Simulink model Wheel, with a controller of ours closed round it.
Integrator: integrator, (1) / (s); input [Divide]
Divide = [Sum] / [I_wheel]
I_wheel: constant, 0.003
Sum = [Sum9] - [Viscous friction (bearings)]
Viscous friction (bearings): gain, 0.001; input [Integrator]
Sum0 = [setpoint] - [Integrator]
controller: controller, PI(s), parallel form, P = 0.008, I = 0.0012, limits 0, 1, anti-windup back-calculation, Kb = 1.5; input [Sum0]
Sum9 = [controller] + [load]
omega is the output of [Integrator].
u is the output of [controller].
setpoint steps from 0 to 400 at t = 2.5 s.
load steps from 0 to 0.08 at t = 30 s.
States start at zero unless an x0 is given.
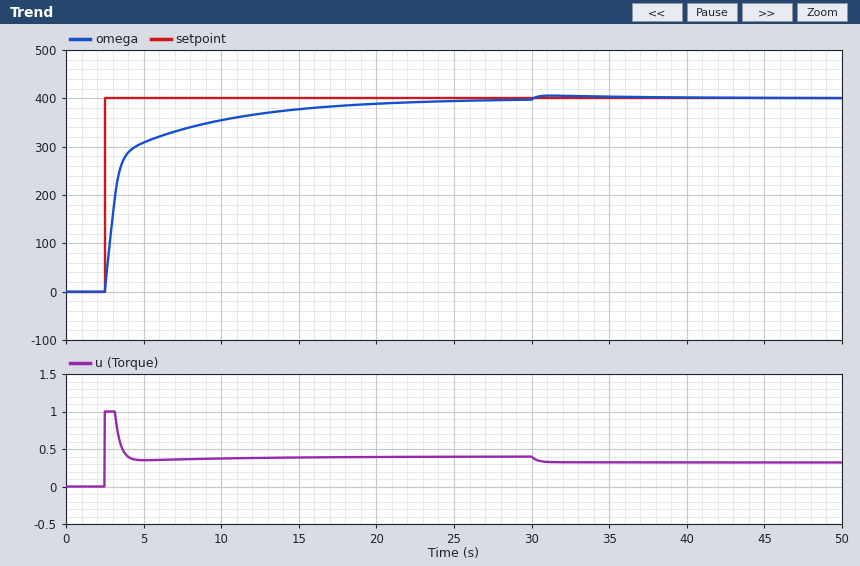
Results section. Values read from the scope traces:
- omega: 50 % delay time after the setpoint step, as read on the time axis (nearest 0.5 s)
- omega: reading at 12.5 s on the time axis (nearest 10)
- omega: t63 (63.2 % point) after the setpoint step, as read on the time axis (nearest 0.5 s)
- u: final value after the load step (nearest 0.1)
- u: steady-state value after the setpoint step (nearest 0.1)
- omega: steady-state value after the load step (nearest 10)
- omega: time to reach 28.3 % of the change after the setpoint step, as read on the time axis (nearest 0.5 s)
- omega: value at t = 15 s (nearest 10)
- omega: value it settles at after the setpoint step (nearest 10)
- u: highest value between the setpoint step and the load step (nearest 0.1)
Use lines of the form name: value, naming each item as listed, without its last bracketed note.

omega: 50 % delay time after the setpoint step, as read on the time axis: 3.0 s
omega: reading at 12.5 s on the time axis: 370
omega: t63 (63.2 % point) after the setpoint step, as read on the time axis: 3.5 s
u: final value after the load step: 0.3
u: steady-state value after the setpoint step: 0.4
omega: steady-state value after the load step: 400
omega: time to reach 28.3 % of the change after the setpoint step, as read on the time axis: 3.0 s
omega: value at t = 15 s: 380
omega: value it settles at after the setpoint step: 400
u: highest value between the setpoint step and the load step: 1.0
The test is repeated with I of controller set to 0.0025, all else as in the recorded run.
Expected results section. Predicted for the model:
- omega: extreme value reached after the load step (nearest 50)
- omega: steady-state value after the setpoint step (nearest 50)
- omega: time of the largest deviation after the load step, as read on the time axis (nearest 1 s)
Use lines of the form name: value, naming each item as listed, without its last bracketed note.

omega: extreme value reached after the load step: 400
omega: steady-state value after the setpoint step: 400
omega: time of the largest deviation after the load step, as read on the time axis: 31 s
